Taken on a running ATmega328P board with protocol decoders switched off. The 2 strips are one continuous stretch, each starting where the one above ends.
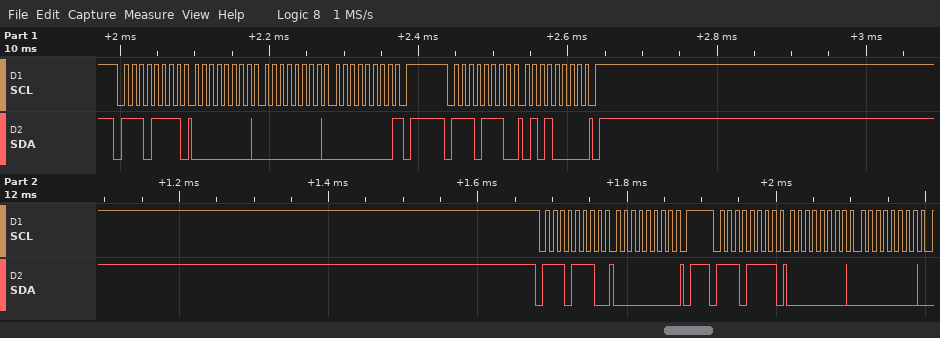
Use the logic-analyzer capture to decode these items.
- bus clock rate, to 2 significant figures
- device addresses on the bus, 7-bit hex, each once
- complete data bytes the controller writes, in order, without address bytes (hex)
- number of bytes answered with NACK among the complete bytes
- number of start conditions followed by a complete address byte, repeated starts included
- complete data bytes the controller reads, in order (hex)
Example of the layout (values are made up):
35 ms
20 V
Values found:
100 kHz
0x77
50 00
1
4
00 00 00 00 00
